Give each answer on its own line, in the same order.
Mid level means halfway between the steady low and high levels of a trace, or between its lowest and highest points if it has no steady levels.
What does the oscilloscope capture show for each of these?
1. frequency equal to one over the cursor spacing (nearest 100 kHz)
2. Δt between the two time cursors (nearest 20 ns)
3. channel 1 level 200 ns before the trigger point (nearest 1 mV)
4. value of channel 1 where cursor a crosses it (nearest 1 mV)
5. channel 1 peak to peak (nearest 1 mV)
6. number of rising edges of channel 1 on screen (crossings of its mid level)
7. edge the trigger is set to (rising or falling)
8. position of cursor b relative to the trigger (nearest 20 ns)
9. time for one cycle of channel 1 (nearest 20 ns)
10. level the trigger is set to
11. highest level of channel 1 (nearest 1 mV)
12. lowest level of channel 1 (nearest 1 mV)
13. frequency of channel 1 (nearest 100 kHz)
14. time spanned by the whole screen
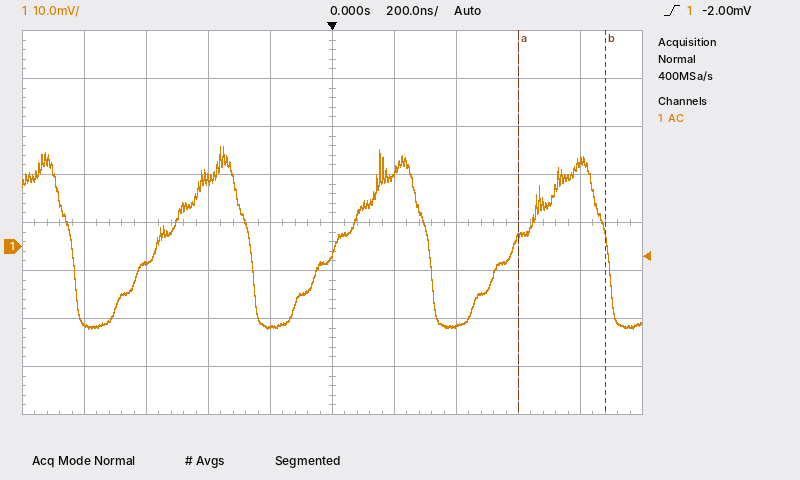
3.6 MHz
280 ns
-17 mV
2 mV
38 mV
3
rising
+880 ns
580 ns
-2.00 mV
21 mV
-17 mV
1.7 MHz
2 µs
